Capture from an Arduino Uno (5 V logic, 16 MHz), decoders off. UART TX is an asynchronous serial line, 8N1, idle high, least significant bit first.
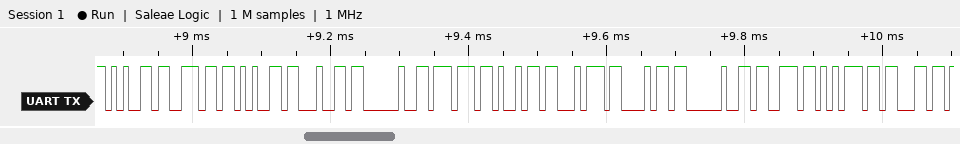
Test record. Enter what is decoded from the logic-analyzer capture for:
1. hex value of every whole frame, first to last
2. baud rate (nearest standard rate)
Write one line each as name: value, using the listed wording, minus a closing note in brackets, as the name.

hex value of every whole frame, first to last: 0x65 0x6E 0x65 0x64 0x20 0x77 0x69 0x74 0x68 0x20 0x73 0x75 0x63
baud rate: 115200 baud
